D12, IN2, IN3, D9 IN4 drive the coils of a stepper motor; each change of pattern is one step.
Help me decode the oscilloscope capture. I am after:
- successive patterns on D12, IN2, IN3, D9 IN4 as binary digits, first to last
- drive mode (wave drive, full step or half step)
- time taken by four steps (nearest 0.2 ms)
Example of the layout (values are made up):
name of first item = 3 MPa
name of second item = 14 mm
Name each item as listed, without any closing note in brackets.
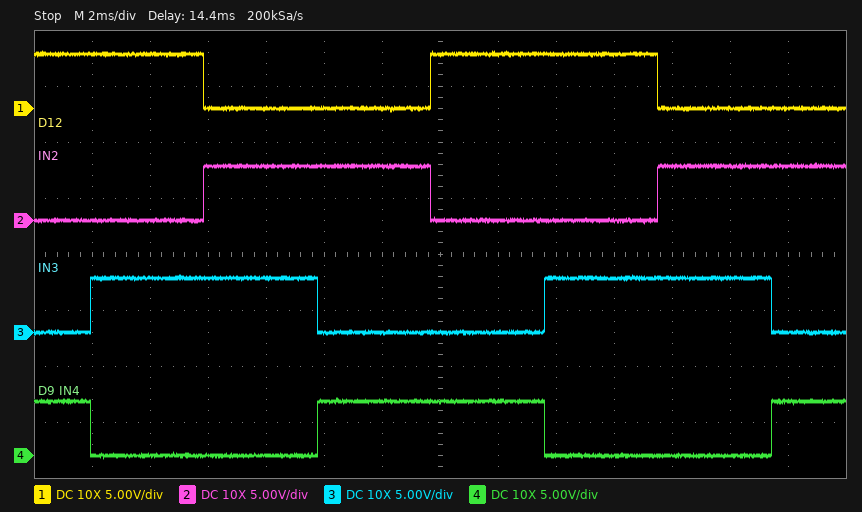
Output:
successive patterns on D12, IN2, IN3, D9 IN4 as binary digits, first to last = 1001 1010 0110 0101 1001 1010 0110 0101
drive mode = full step
time taken by four steps = 15.6 ms
